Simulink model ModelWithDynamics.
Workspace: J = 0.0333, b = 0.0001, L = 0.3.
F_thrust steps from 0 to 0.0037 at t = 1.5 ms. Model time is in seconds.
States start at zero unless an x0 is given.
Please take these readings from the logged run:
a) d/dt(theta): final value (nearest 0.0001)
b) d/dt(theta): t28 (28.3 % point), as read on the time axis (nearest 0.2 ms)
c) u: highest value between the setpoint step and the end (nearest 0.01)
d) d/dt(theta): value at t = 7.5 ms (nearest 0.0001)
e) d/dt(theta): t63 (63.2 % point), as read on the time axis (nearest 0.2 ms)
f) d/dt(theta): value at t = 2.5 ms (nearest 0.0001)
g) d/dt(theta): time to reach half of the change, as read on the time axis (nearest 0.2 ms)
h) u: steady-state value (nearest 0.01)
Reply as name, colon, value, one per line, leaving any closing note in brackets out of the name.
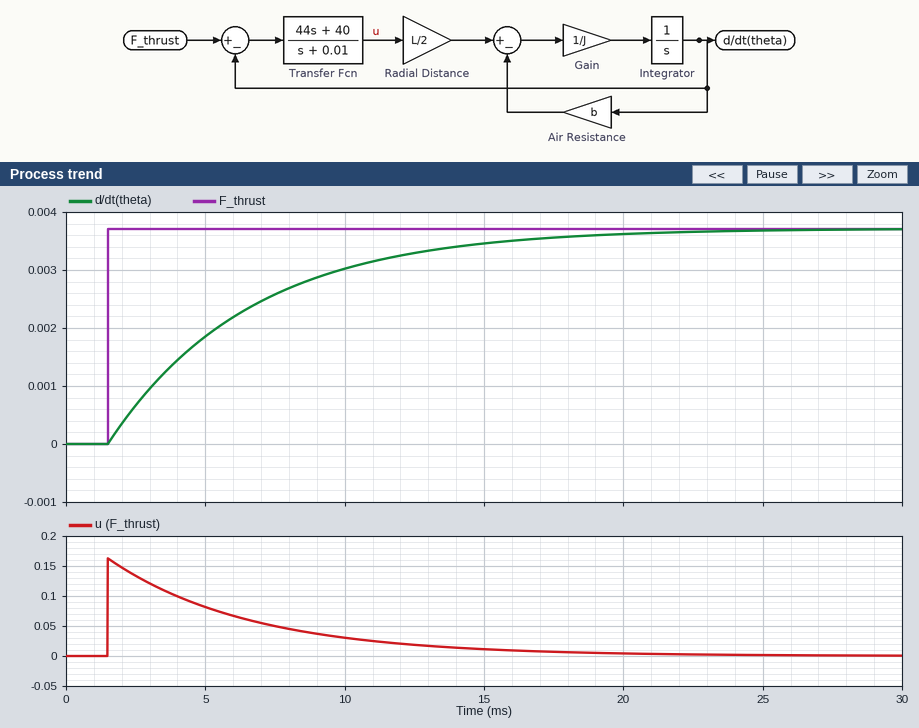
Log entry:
d/dt(theta): final value: 0.0037
d/dt(theta): t28 (28.3 % point), as read on the time axis: 3.2 ms
u: highest value between the setpoint step and the end: 0.16
d/dt(theta): value at t = 7.5 ms: 0.0026
d/dt(theta): t63 (63.2 % point), as read on the time axis: 6.6 ms
d/dt(theta): value at t = 2.5 ms: 0.0007
d/dt(theta): time to reach half of the change, as read on the time axis: 5.0 ms
u: steady-state value: 0.00
